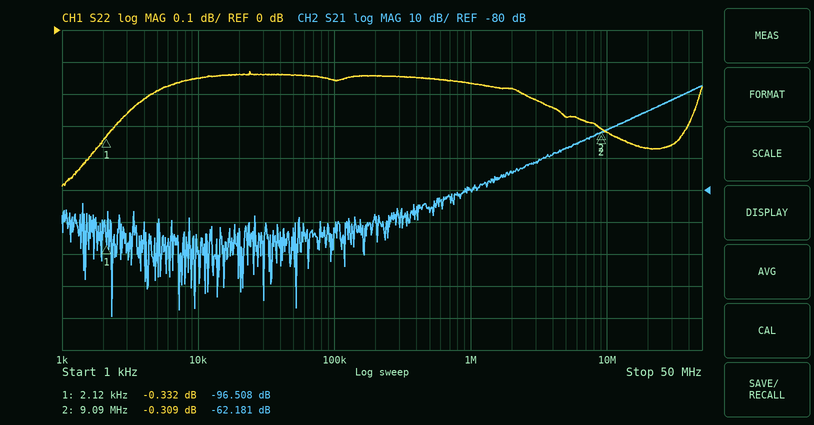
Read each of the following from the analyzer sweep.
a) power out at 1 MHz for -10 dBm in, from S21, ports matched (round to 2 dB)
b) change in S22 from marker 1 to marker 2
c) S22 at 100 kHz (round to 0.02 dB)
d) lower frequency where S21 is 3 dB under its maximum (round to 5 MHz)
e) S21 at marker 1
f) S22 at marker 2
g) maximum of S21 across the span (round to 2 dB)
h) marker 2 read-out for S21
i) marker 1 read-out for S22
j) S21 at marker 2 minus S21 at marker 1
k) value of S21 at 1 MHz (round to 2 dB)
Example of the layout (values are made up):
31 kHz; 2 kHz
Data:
-90 dBm; 0.023 dB; -0.16 dB; 35 MHz; -96.508 dB; -0.309 dB; -48 dB; -62.181 dB; -0.332 dB; 34.327 dB; -80 dB
